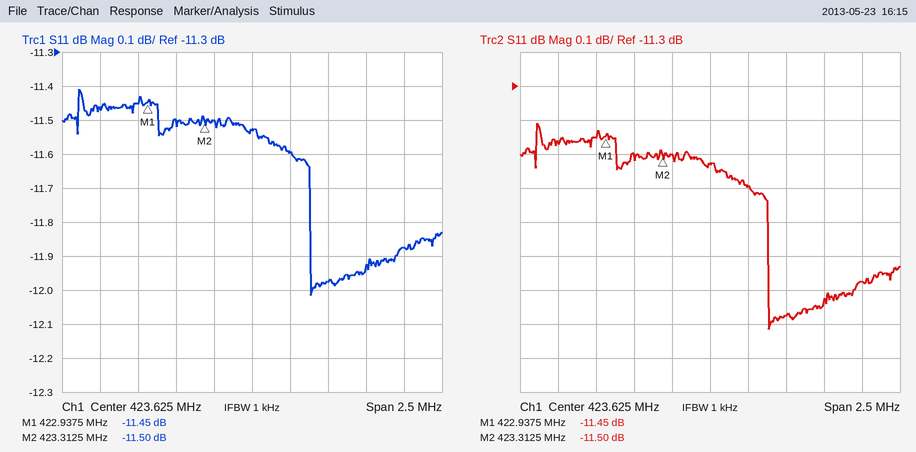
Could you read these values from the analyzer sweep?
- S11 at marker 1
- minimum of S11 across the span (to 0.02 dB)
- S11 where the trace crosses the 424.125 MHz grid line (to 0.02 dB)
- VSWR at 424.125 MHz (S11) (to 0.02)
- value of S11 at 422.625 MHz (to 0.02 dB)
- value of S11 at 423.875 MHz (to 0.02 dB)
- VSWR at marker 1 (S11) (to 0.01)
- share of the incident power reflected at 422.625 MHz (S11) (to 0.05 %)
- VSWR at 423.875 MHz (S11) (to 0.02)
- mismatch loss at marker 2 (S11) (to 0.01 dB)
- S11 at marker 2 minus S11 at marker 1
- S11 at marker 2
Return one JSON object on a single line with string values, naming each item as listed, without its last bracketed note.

{"S11 at marker 1": "-11.45 dB", "minimum of S11 across the span": "-12.02 dB", "S11 where the trace crosses the 424.125 MHz grid line": "-11.98 dB", "VSWR at 424.125 MHz (S11)": "1.68", "value of S11 at 422.625 MHz": "-11.46 dB", "value of S11 at 423.875 MHz": "-11.60 dB", "VSWR at marker 1 (S11)": "1.73", "share of the incident power reflected at 422.625 MHz (S11)": "7.15 %", "VSWR at 423.875 MHz (S11)": "1.72", "mismatch loss at marker 2 (S11)": "0.32 dB", "S11 at marker 2 minus S11 at marker 1": "-0.05 dB", "S11 at marker 2": "-11.50 dB"}
